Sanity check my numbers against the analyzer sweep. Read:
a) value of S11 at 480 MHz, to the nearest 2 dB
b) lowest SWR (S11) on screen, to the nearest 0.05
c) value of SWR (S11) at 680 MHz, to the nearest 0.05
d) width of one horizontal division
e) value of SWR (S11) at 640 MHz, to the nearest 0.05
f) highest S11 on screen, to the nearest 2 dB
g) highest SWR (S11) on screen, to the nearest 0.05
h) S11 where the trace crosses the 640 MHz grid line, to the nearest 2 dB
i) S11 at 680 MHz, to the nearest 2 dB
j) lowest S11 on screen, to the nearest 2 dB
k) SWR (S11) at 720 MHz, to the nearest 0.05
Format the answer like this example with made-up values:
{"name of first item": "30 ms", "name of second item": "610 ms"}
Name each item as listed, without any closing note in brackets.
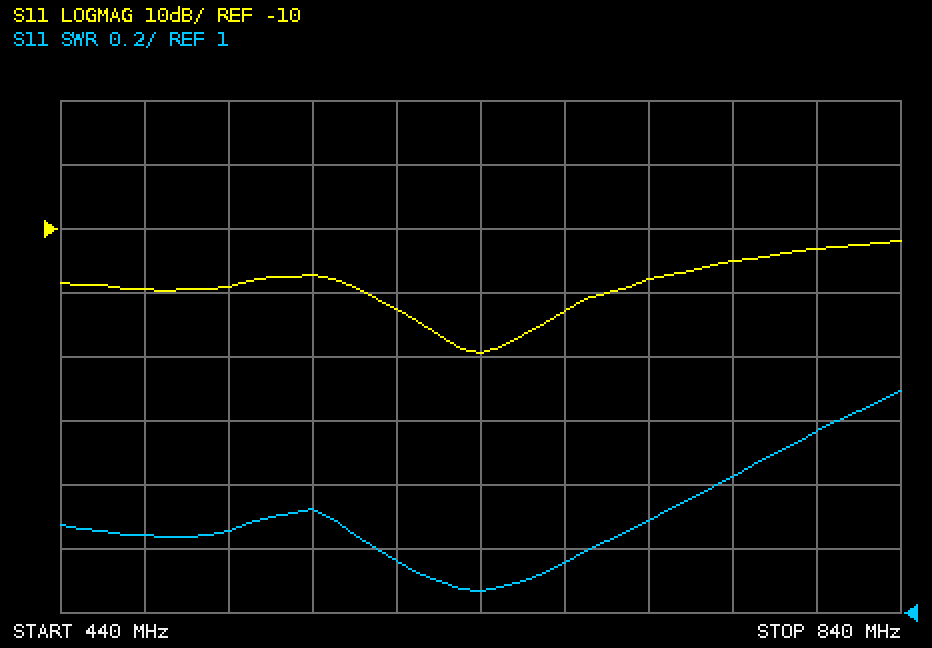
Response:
{"value of S11 at 480 MHz, to the nearest 2 dB": "-20 dB", "lowest SWR (S11) on screen, to the nearest 0.05": "1.05", "value of SWR (S11) at 680 MHz, to the nearest 0.05": "1.15", "width of one horizontal division": "40 MHz", "value of SWR (S11) at 640 MHz, to the nearest 0.05": "1.05", "highest S11 on screen, to the nearest 2 dB": "-12 dB", "highest SWR (S11) on screen, to the nearest 0.05": "1.70", "S11 where the trace crosses the 640 MHz grid line, to the nearest 2 dB": "-30 dB", "S11 at 680 MHz, to the nearest 2 dB": "-22 dB", "lowest S11 on screen, to the nearest 2 dB": "-30 dB", "SWR (S11) at 720 MHz, to the nearest 0.05": "1.30"}
